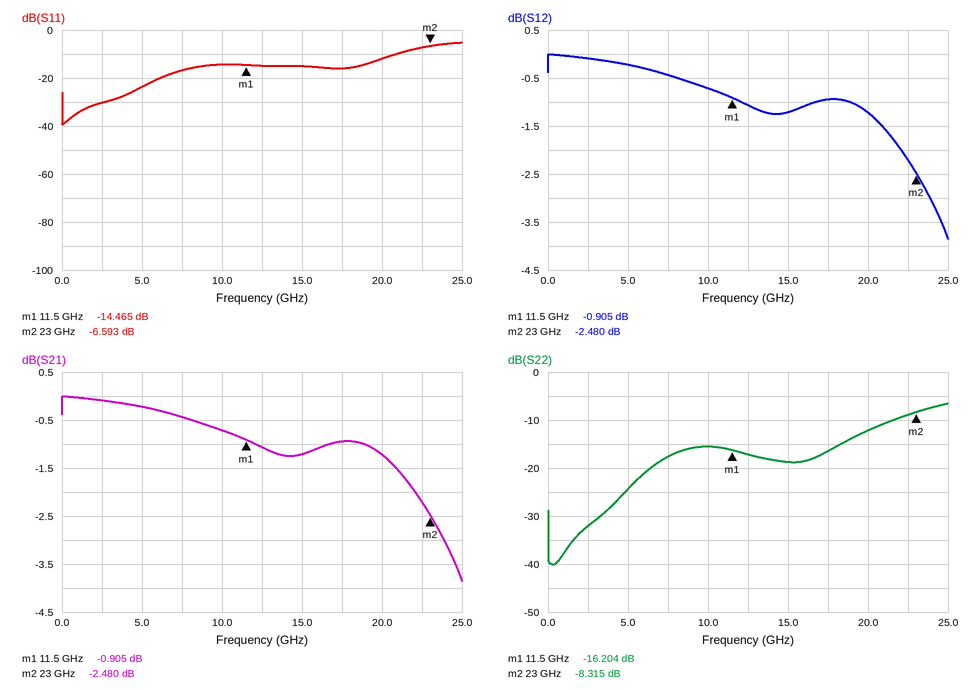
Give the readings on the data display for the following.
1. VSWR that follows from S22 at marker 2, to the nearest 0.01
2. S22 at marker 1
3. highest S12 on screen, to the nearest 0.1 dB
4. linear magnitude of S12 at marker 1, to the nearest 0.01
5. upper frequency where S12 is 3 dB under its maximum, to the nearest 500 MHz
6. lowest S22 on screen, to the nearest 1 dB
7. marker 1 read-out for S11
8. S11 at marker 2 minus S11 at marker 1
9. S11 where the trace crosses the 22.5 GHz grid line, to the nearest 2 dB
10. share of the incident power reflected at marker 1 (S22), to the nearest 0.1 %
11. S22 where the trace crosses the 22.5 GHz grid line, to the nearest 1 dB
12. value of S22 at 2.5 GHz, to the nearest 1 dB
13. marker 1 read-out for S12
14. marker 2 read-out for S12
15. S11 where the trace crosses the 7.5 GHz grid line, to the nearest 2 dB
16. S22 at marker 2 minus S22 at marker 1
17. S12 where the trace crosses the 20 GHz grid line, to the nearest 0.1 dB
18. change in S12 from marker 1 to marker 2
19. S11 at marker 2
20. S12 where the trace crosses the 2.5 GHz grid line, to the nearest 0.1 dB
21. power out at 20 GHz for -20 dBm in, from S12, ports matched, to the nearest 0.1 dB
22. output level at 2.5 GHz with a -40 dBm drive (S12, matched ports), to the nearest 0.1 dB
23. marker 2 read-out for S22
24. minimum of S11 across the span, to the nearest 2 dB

2.25
-16.204 dB
0.0 dB
0.90
24.0 GHz
-40 dB
-14.465 dB
7.872 dB
-8 dB
2.4 %
-9 dB
-32 dB
-0.905 dB
-2.480 dB
-16 dB
7.889 dB
-1.2 dB
-1.575 dB
-6.593 dB
-0.1 dB
-21.2 dBm
-40.1 dBm
-8.315 dB
-40 dB
